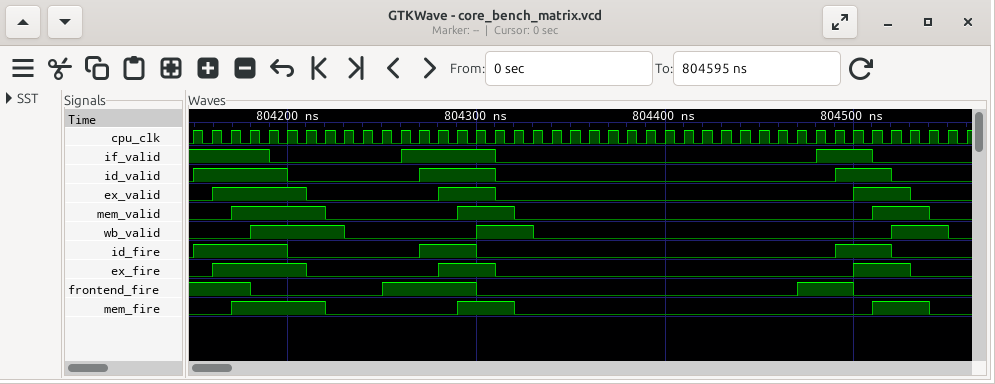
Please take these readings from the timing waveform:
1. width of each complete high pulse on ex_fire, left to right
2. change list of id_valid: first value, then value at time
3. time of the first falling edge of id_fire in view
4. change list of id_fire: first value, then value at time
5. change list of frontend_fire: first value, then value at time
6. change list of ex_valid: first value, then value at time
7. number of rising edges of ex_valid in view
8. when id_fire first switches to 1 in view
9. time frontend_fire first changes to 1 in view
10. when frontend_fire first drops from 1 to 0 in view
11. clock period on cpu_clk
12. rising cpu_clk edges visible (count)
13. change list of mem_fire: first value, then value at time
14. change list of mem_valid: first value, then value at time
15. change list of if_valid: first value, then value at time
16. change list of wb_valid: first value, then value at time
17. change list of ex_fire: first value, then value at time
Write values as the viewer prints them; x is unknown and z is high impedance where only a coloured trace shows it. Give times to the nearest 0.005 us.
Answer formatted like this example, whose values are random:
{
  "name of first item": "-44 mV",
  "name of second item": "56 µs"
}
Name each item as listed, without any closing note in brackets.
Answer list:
{
  "width of each complete high pulse on ex_fire, left to right": "0.05 us, 0.03 us, 0.03 us",
  "change list of id_valid: first value, then value at time": "0, 1 at 804.15 us, 0 at 804.2 us, 1 at 804.27 us, 0 at 804.31 us, 1 at 804.49 us, 0 at 804.52 us",
  "time of the first falling edge of id_fire in view": "804.2 us",
  "change list of id_fire: first value, then value at time": "0, 1 at 804.15 us, 0 at 804.2 us, 1 at 804.27 us, 0 at 804.3 us, 1 at 804.49 us, 0 at 804.52 us",
  "change list of frontend_fire: first value, then value at time": "1, 0 at 804.18 us, 1 at 804.25 us, 0 at 804.3 us, 1 at 804.47 us, 0 at 804.5 us",
  "change list of ex_valid: first value, then value at time": "0, 1 at 804.16 us, 0 at 804.21 us, 1 at 804.28 us, 0 at 804.31 us, 1 at 804.5 us, 0 at 804.53 us",
  "number of rising edges of ex_valid in view": "3",
  "when id_fire first switches to 1 in view": "804.15 us",
  "time frontend_fire first changes to 1 in view": "804.25 us",
  "when frontend_fire first drops from 1 to 0 in view": "804.18 us",
  "clock period on cpu_clk": "0.01 us",
  "rising cpu_clk edges visible": "42",
  "change list of mem_fire: first value, then value at time": "0, 1 at 804.17 us, 0 at 804.22 us, 1 at 804.29 us, 0 at 804.32 us, 1 at 804.51 us, 0 at 804.54 us",
  "change list of mem_valid: first value, then value at time": "0, 1 at 804.17 us, 0 at 804.22 us, 1 at 804.29 us, 0 at 804.32 us, 1 at 804.51 us, 0 at 804.54 us",
  "change list of if_valid: first value, then value at time": "1, 0 at 804.19 us, 1 at 804.26 us, 0 at 804.31 us, 1 at 804.48 us, 0 at 804.51 us",
  "change list of wb_valid: first value, then value at time": "0, 1 at 804.18 us, 0 at 804.23 us, 1 at 804.3 us, 0 at 804.33 us, 1 at 804.52 us, 0 at 804.55 us",
  "change list of ex_fire: first value, then value at time": "0, 1 at 804.16 us, 0 at 804.21 us, 1 at 804.28 us, 0 at 804.31 us, 1 at 804.5 us, 0 at 804.53 us"
}
